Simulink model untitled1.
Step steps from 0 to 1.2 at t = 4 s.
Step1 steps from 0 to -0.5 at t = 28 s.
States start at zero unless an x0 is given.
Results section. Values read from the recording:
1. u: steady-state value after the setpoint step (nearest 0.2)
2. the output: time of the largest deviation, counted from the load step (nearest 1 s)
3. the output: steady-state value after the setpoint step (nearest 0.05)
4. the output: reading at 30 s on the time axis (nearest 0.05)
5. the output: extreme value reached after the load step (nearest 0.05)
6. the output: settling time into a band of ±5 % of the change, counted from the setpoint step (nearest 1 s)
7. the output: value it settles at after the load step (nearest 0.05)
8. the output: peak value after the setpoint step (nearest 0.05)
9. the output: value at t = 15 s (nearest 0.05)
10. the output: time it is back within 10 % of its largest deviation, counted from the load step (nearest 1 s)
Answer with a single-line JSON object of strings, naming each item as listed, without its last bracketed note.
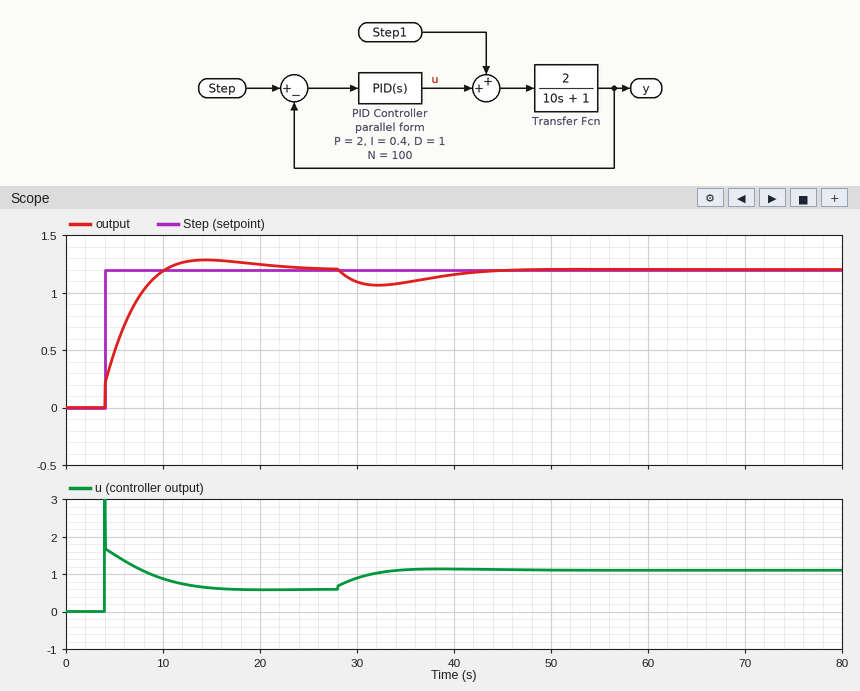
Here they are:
{"u: steady-state value after the setpoint step": "0.6", "the output: time of the largest deviation, counted from the load step": "4 s", "the output: steady-state value after the setpoint step": "1.20", "the output: reading at 30 s on the time axis": "1.10", "the output: extreme value reached after the load step": "1.05", "the output: settling time into a band of ±5 % of the change, counted from the setpoint step": "14 s", "the output: value it settles at after the load step": "1.20", "the output: peak value after the setpoint step": "1.30", "the output: value at t = 15 s": "1.30", "the output: time it is back within 10 % of its largest deviation, counted from the load step": "16 s"}
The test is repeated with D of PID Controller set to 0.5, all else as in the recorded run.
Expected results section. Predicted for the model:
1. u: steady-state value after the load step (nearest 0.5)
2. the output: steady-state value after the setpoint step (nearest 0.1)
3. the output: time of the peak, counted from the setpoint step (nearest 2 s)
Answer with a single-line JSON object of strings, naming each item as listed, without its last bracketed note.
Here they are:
{"u: steady-state value after the load step": "1.0", "the output: steady-state value after the setpoint step": "1.2", "the output: time of the peak, counted from the setpoint step": "10 s"}
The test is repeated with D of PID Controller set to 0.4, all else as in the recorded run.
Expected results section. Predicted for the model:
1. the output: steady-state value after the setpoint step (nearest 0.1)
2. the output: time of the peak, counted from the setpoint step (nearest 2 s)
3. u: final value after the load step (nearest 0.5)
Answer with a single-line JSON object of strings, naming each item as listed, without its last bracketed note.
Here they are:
{"the output: steady-state value after the setpoint step": "1.2", "the output: time of the peak, counted from the setpoint step": "10 s", "u: final value after the load step": "1.0"}
